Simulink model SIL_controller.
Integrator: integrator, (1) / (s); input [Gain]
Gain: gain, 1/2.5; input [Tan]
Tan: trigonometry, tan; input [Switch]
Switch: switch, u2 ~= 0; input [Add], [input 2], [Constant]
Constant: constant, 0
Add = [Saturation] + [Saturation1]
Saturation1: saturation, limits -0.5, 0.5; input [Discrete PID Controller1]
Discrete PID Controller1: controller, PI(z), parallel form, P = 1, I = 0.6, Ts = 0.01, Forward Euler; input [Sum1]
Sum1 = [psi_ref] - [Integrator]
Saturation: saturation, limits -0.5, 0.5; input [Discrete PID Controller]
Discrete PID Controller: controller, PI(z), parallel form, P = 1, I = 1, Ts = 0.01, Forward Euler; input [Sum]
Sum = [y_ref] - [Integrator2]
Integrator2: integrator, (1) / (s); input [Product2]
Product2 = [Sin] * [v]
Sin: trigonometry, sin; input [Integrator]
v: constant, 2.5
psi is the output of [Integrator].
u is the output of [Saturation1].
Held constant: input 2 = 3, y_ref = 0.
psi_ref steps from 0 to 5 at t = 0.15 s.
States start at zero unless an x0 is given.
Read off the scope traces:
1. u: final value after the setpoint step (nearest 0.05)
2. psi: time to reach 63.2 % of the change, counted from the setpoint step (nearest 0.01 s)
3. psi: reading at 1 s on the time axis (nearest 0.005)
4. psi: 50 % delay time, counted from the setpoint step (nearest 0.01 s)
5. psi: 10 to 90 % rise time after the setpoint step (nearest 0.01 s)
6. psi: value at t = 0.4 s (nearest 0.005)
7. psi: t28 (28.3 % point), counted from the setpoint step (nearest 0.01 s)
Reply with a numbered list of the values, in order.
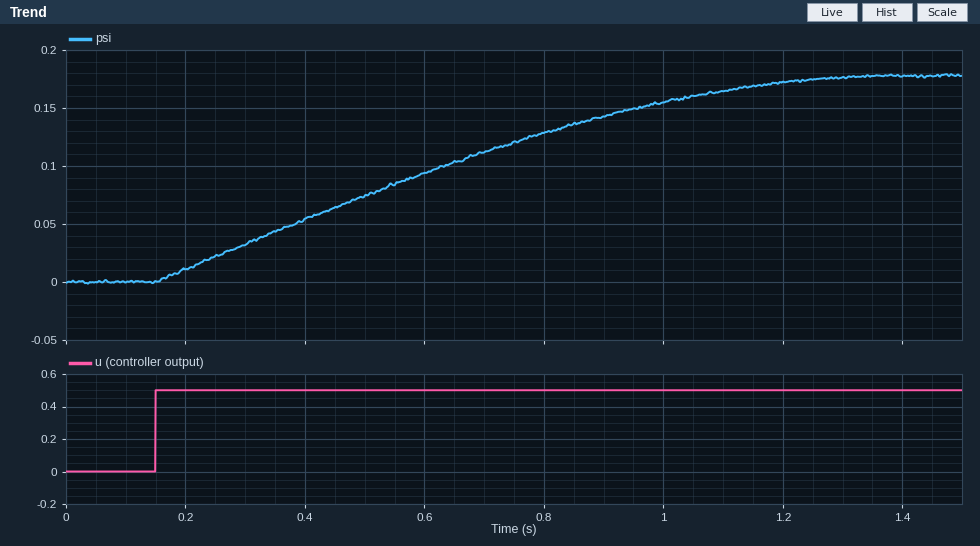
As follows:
1. 0.50
2. 0.55 s
3. 0.155
4. 0.42 s
5. 0.82 s
6. 0.055
7. 0.23 s
